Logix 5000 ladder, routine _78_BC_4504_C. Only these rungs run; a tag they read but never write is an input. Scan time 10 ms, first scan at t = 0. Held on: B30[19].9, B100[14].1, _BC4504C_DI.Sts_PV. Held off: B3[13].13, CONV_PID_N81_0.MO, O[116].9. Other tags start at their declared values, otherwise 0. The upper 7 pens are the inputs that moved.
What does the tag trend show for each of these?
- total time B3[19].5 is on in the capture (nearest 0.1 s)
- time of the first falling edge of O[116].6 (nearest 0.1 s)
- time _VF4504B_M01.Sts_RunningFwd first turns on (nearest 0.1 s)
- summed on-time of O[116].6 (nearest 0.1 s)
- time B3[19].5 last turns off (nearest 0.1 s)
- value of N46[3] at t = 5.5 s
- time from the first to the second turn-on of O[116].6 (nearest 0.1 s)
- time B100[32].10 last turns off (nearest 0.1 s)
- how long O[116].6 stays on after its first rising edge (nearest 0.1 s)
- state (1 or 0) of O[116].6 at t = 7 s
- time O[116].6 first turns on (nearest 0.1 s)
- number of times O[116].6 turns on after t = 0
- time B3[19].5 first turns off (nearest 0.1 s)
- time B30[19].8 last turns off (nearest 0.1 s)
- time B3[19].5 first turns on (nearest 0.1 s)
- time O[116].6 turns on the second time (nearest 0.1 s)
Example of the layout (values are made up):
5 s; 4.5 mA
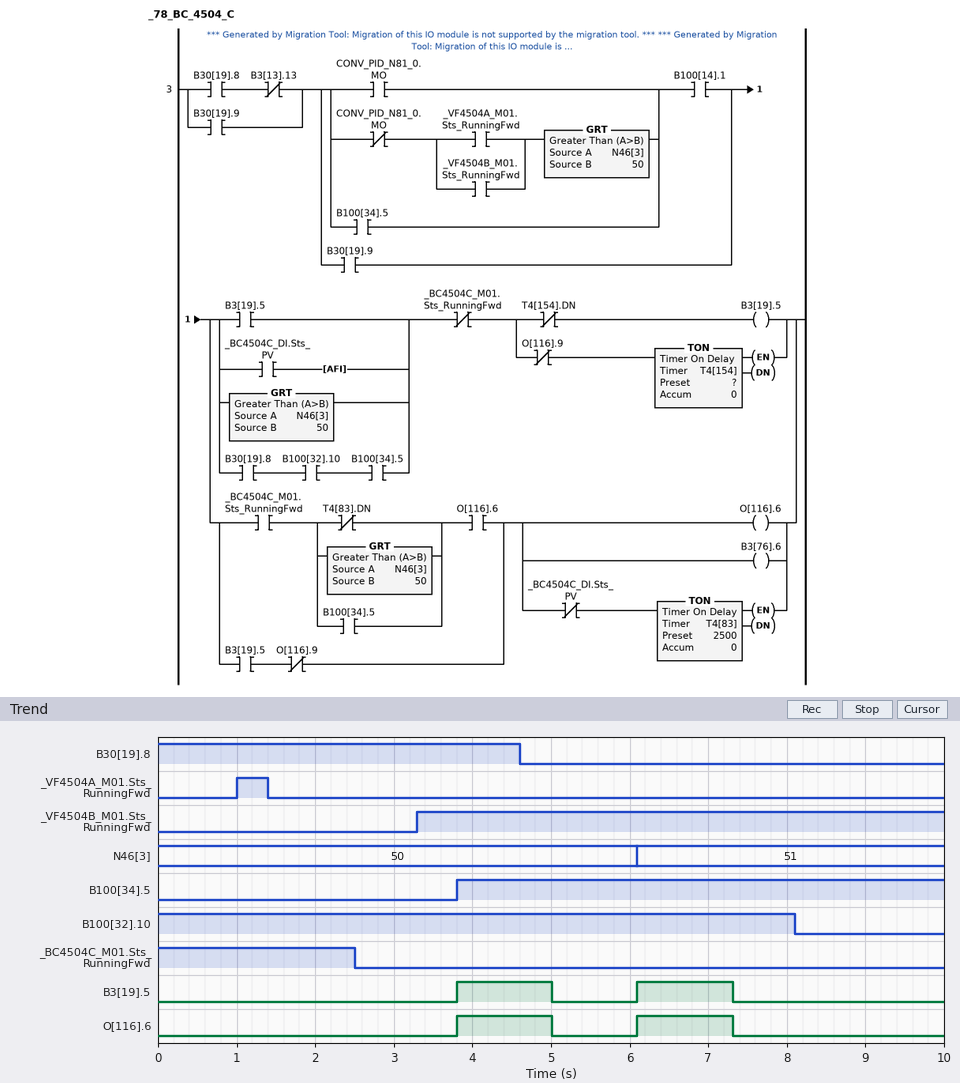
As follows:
2.4 s; 5.0 s; 3.3 s; 2.4 s; 7.3 s; 50; 2.3 s; 8.1 s; 1.2 s; 1; 3.8 s; 2; 5.0 s; 4.6 s; 3.8 s; 6.1 s
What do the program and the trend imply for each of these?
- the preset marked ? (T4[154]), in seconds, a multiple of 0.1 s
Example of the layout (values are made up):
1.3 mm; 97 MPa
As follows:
1.2 s
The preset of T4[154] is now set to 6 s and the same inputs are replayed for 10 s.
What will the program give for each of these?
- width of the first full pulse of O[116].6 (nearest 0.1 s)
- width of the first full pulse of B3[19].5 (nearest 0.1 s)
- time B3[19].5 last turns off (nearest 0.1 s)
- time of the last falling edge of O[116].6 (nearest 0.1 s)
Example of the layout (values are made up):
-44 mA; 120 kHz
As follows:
6.0 s; 6.0 s; 9.8 s; 9.8 s
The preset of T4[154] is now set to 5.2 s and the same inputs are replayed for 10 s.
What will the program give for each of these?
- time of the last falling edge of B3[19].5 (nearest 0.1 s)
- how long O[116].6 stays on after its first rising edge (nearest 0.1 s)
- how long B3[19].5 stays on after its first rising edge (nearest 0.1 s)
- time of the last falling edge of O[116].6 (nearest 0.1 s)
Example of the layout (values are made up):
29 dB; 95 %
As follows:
9.0 s; 5.2 s; 5.2 s; 9.0 s
